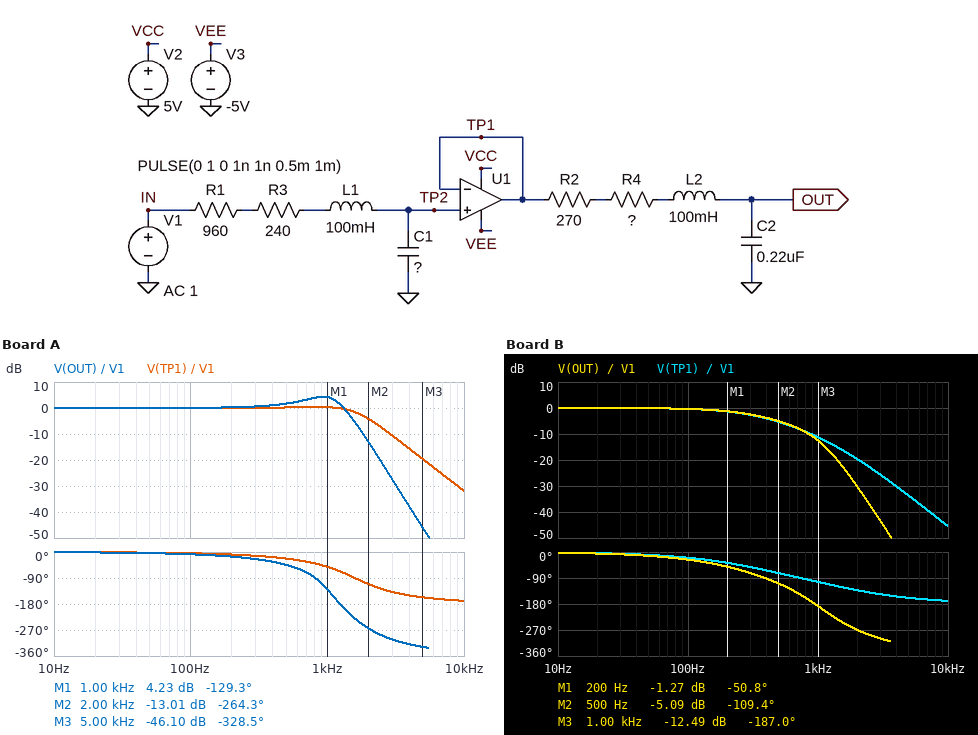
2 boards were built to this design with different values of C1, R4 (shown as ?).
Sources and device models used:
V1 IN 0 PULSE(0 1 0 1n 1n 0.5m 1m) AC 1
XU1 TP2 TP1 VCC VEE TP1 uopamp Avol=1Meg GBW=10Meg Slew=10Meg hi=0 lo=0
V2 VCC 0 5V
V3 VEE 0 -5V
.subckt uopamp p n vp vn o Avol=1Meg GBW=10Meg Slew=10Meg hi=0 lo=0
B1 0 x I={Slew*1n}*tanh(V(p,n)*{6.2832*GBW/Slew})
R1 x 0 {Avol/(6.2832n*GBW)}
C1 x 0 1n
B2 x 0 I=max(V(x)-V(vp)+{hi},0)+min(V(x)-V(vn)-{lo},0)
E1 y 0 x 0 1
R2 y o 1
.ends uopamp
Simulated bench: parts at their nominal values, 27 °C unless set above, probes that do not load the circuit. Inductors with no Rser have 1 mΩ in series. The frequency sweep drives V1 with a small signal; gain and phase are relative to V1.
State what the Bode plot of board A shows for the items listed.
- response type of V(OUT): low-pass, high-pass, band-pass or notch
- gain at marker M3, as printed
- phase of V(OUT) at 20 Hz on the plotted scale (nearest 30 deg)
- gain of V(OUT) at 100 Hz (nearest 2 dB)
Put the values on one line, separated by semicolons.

low-pass; -46.10 dB; 0 deg; 0 dB
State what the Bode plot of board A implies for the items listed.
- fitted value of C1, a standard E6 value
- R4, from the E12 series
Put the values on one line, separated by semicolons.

100 nF; 180 Ω
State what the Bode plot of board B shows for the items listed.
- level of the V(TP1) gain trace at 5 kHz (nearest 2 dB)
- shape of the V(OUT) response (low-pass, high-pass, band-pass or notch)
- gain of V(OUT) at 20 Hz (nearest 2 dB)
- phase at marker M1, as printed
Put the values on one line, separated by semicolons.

-34 dB; low-pass; 0 dB; -50.8 deg
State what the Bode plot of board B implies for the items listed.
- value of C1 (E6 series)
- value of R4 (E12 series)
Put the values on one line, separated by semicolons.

470 nF; 560 Ω
